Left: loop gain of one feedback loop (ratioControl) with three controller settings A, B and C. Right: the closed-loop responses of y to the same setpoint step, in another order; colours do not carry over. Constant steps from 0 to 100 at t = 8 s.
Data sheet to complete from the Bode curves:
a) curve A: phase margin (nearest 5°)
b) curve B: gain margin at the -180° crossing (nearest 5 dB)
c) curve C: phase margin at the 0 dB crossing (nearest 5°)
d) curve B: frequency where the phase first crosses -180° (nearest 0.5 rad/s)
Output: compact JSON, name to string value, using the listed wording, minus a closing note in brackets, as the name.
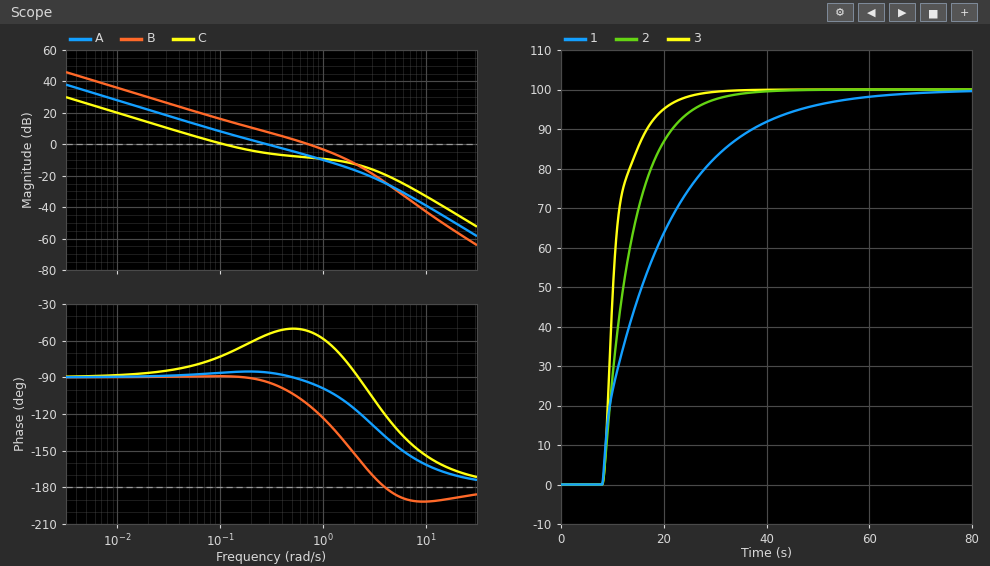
{"curve A: phase margin": "95°", "curve B: gain margin at the -180° crossing": "25 dB", "curve C: phase margin at the 0 dB crossing": "110°", "curve B: frequency where the phase first crosses -180°": "4.0 rad/s"}
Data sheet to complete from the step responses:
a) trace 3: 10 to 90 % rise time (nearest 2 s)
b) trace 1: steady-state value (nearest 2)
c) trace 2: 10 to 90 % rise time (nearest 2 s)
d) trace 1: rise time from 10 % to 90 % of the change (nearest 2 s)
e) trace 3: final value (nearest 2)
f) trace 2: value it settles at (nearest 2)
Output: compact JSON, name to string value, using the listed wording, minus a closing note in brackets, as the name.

{"trace 3: 10 to 90 % rise time": "8 s", "trace 1: steady-state value": "100", "trace 2: 10 to 90 % rise time": "12 s", "trace 1: rise time from 10 % to 90 % of the change": "28 s", "trace 3: final value": "100", "trace 2: value it settles at": "100"}
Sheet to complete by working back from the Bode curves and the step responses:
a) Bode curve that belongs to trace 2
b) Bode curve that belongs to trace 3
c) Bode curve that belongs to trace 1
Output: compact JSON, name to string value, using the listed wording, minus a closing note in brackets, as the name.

{"Bode curve that belongs to trace 2": "A", "Bode curve that belongs to trace 3": "B", "Bode curve that belongs to trace 1": "C"}
